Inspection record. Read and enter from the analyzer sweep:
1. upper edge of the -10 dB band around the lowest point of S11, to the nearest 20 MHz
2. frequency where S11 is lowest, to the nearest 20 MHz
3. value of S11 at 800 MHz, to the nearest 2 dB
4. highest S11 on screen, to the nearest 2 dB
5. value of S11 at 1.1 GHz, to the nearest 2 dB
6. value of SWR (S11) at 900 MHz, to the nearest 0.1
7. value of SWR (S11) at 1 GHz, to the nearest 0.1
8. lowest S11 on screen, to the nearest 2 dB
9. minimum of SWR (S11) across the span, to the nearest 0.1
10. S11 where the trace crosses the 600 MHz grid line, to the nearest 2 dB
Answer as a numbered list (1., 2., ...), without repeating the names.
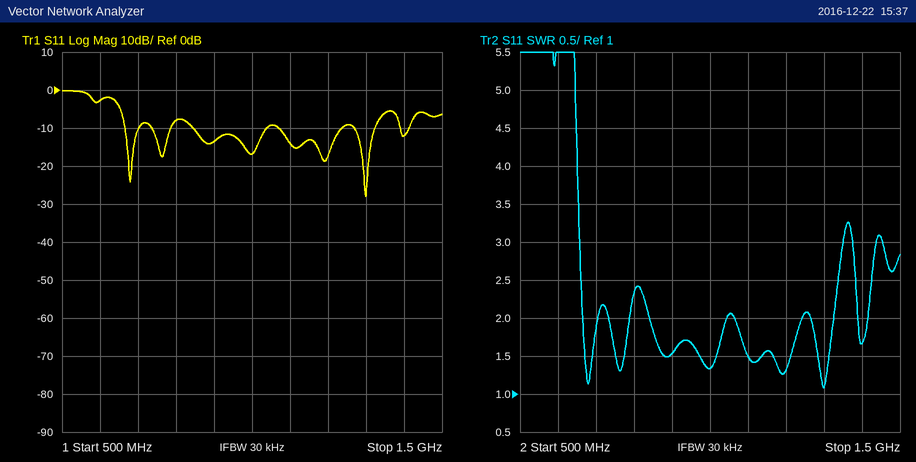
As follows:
1. 1.32 GHz
2. 1.30 GHz
3. -8 dB
4. 0 dB
5. -14 dB
6. 1.5
7. 1.3
8. -28 dB
9. 1.1
10. -2 dB
